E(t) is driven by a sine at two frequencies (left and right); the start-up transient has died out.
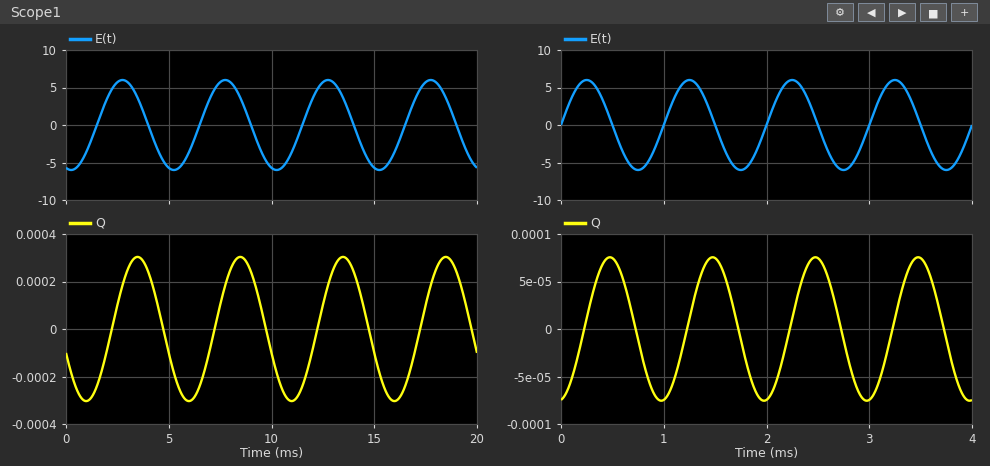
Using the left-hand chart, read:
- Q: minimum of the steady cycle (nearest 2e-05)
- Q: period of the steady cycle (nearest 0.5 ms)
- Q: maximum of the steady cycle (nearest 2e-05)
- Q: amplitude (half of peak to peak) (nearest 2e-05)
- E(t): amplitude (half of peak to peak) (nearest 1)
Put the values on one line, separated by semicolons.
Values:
-0.00030; 5.0 ms; 0.00030; 0.00030; 6
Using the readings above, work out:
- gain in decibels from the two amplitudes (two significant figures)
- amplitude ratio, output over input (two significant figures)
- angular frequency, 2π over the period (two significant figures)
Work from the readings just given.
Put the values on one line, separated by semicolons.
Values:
-86 dB; 0.000050; 1.3 rad/ms
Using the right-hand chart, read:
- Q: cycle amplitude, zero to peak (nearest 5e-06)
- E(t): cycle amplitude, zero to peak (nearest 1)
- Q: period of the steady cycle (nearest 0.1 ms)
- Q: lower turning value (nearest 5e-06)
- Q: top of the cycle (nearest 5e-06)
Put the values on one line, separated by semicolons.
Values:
0.000075; 6; 1.0 ms; -0.000075; 0.000075
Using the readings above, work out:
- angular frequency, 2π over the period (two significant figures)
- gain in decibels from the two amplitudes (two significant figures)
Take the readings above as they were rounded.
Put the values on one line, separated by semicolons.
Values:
6.3 rad/ms; -98 dB
